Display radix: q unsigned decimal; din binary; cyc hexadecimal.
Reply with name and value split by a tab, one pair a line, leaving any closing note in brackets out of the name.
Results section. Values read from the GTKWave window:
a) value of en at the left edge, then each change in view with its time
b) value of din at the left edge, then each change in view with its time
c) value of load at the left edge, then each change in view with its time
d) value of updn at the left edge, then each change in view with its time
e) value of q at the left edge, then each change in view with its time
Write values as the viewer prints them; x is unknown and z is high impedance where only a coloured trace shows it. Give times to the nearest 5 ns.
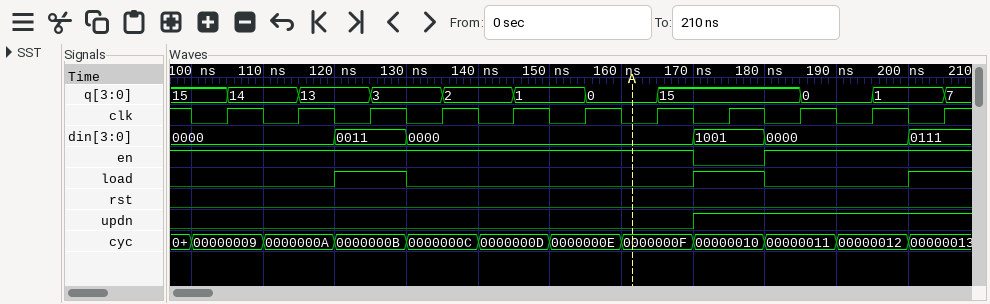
value of en at the left edge, then each change in view with its time	1, 0 at 170 ns, 1 at 180 ns
value of din at the left edge, then each change in view with its time	0000, 0011 at 120 ns, 0000 at 130 ns, 1001 at 170 ns, 0000 at 180 ns, 0111 at 200 ns
value of load at the left edge, then each change in view with its time	0, 1 at 120 ns, 0 at 130 ns, 1 at 170 ns, 0 at 180 ns, 1 at 200 ns
value of updn at the left edge, then each change in view with its time	0, 1 at 170 ns
value of q at the left edge, then each change in view with its time	15, 14 at 105 ns, 13 at 115 ns, 3 at 125 ns, 2 at 135 ns, 1 at 145 ns, 0 at 155 ns, 15 at 165 ns, 0 at 185 ns, 1 at 195 ns, 7 at 205 ns
